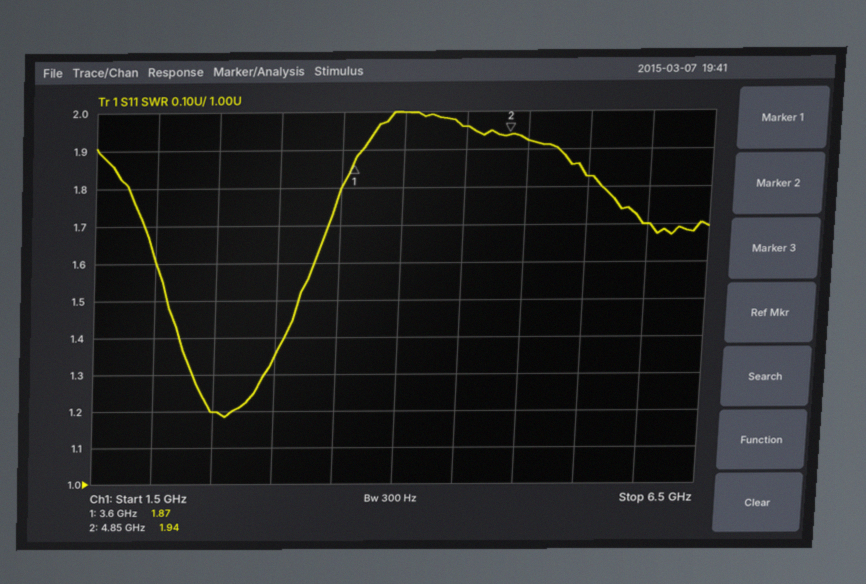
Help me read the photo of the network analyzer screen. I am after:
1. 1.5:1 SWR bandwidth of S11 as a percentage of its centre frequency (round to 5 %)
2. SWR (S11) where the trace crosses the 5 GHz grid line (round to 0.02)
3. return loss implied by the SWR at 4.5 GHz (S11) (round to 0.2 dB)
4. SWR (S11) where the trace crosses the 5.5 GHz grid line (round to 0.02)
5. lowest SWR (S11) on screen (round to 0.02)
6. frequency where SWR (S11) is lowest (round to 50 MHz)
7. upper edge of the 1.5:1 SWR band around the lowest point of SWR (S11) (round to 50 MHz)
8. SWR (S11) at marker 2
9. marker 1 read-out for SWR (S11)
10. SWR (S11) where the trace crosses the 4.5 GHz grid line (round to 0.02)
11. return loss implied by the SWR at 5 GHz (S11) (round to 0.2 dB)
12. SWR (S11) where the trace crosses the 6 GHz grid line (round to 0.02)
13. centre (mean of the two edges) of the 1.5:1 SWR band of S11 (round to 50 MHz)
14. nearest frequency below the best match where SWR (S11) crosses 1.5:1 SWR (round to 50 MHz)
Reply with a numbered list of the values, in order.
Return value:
1. 40 %
2. 1.92
3. 9.8 dB
4. 1.82
5. 1.18
6. 2.60 GHz
7. 3.20 GHz
8. 1.94
9. 1.87
10. 1.96
11. 10.0 dB
12. 1.70
13. 2.65 GHz
14. 2.10 GHz
